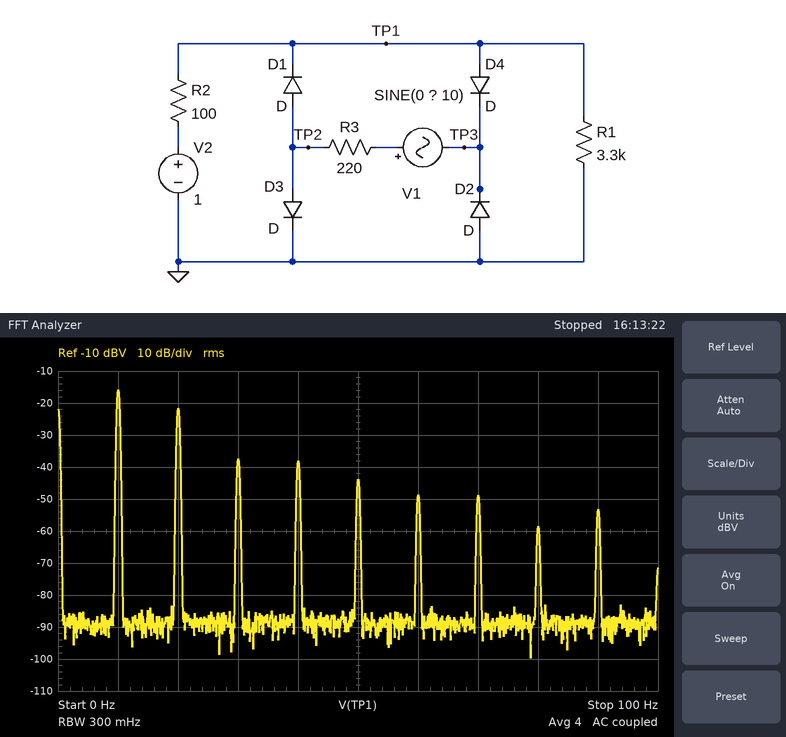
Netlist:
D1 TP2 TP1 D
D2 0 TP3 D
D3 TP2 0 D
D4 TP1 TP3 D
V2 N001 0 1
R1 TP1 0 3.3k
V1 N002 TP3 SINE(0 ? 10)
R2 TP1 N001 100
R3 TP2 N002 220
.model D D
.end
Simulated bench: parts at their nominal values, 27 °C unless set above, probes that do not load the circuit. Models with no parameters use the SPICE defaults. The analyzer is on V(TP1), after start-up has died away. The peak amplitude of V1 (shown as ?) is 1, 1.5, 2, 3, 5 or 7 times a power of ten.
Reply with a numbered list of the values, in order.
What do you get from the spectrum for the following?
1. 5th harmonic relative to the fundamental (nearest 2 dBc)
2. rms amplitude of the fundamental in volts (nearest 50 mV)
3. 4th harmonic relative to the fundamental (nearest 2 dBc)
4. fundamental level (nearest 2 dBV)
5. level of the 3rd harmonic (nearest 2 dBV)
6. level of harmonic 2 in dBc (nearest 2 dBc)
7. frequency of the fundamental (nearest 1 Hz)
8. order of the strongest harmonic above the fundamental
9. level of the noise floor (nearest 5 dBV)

1. -28 dBc
2. 150 mV
3. -22 dBc
4. -16 dBV
5. -38 dBV
6. -6 dBc
7. 10 Hz
8. 2
9. -90 dBV
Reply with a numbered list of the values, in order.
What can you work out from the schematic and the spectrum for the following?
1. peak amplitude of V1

1. 2 V
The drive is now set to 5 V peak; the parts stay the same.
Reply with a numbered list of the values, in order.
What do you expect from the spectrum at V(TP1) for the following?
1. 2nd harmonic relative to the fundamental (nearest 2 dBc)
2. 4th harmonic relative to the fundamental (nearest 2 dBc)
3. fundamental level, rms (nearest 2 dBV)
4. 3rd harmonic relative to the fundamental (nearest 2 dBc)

1. -8 dBc
2. -14 dBc
3. -8 dBV
4. -20 dBc
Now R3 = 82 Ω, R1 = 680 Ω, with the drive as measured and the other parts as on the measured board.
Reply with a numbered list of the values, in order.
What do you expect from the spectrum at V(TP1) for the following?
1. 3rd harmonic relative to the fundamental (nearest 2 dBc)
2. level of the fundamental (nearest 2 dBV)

1. -18 dBc
2. -12 dBV
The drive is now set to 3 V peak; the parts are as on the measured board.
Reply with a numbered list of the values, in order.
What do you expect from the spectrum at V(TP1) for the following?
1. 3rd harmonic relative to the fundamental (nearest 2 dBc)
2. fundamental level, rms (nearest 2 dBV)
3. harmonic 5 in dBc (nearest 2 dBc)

1. -24 dBc
2. -12 dBV
3. -30 dBc
